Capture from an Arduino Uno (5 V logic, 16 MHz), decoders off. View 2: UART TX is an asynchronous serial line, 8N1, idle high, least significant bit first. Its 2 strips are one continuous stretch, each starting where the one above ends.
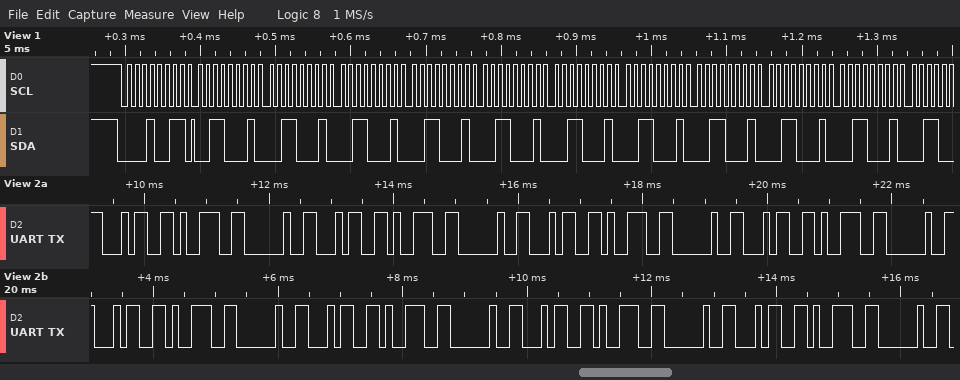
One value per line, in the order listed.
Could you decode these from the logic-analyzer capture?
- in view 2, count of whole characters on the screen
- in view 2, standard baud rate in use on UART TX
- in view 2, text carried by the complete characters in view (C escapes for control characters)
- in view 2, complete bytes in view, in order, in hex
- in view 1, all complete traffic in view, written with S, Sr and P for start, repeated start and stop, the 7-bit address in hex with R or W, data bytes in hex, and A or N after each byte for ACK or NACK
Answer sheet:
24
9600 baud
"49 49 49 49 49 49 49 49 "
34 39 20 34 39 20 34 39 20 34 39 20 34 39 20 34 39 20 34 39 20 34 39 20
S 09R A 31 A 31 A 31 A 31 A 31 A 31 A 31 A 31 A 31 A 31 A
